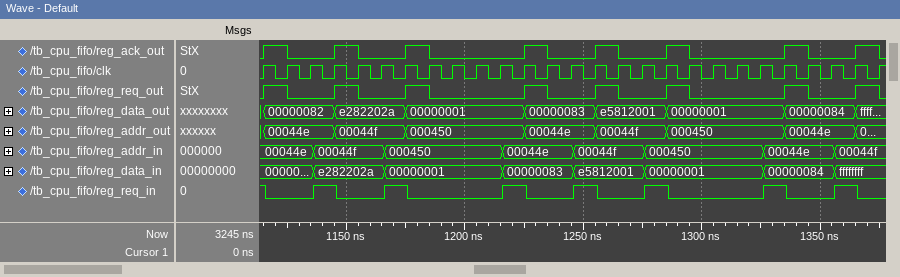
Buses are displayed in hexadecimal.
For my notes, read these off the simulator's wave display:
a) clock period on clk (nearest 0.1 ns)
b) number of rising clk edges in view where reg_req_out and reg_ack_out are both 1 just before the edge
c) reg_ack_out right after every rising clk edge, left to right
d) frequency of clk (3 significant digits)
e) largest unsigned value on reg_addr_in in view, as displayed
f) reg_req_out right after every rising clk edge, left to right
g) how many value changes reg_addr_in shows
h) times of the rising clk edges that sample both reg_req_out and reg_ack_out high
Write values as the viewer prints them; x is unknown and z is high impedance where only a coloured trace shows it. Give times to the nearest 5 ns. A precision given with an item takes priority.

10 ns
8
1 0 0 1 0 0 1 0 0 0 0 1 0 0 1 0 0 1 0 0 0 0 1 0 0 1 0
100 MHz
000450
1 0 0 1 0 0 1 0 0 0 0 1 0 0 1 0 0 1 0 0 0 0 1 0 0 1 0
7
1125 ns, 1155 ns, 1185 ns, 1235 ns, 1265 ns, 1295 ns, 1345 ns, 1375 ns
